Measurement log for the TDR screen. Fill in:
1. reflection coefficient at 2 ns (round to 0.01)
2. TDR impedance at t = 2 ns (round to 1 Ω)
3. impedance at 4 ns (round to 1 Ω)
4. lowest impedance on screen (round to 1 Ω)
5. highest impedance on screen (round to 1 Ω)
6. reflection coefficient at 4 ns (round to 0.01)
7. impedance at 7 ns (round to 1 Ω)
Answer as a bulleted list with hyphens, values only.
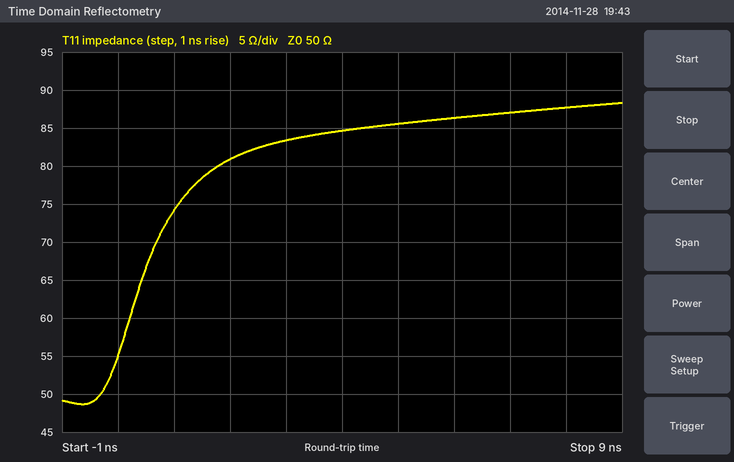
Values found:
- +0.24
- 81 Ω
- 85 Ω
- 49 Ω
- 88 Ω
- +0.26
- 87 Ω
